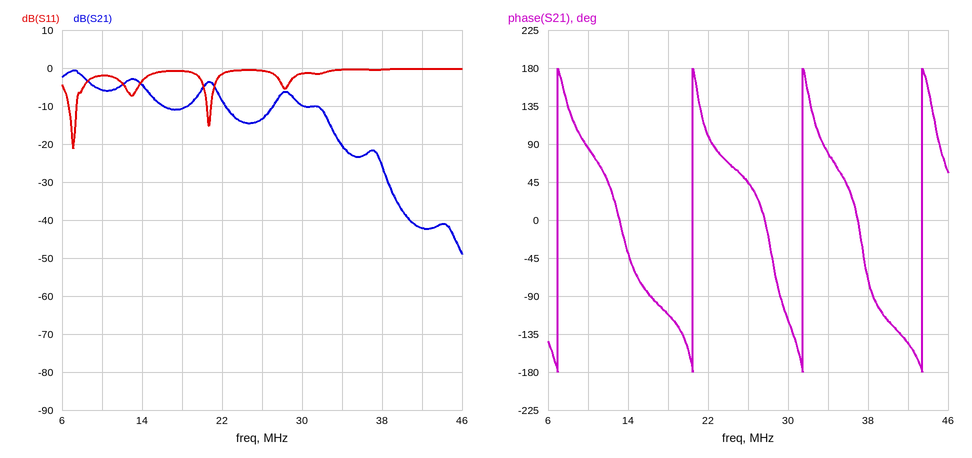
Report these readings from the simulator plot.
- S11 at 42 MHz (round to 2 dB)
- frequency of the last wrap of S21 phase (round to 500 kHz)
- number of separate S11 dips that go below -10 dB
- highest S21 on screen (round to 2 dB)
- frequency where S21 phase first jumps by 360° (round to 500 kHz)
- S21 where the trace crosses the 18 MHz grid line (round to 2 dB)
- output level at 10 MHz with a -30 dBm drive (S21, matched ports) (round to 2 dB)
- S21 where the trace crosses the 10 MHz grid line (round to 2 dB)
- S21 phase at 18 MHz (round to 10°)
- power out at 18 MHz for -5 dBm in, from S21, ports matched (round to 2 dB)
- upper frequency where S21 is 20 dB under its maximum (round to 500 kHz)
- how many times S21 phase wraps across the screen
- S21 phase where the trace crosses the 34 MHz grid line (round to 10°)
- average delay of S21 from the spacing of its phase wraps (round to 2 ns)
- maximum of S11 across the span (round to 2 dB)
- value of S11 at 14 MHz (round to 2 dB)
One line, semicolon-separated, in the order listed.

0 dB; 43.5 MHz; 2; 0 dB; 7.0 MHz; -10 dB; -36 dBm; -6 dB; -110°; -16 dBm; 34.0 MHz; 4; 80°; 82 ns; 0 dB; -4 dB
